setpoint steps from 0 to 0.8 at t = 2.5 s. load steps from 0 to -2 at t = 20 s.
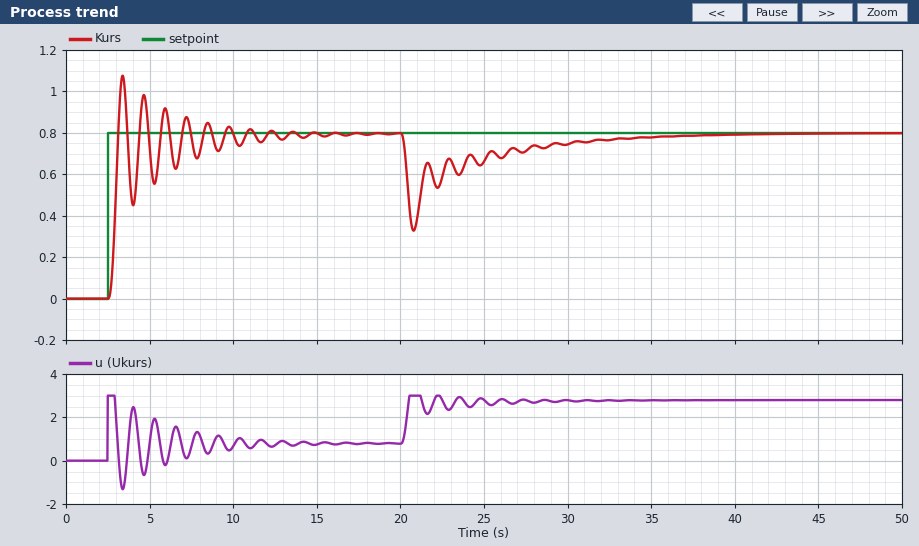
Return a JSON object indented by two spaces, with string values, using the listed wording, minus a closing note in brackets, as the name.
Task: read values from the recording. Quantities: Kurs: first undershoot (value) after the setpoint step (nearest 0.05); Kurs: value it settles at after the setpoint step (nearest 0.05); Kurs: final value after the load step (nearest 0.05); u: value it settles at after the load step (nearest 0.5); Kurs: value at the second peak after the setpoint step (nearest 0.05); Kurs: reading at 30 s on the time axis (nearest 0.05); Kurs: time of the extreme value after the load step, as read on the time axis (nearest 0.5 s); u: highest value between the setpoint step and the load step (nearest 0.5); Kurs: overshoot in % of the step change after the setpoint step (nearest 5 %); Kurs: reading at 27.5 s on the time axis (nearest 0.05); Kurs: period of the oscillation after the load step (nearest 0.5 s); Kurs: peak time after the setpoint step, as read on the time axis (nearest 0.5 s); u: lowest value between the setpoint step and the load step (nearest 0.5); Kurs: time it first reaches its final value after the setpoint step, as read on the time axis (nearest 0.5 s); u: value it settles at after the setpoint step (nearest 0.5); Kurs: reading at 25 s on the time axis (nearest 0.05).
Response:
{
  "Kurs: first undershoot (value) after the setpoint step": "0.45",
  "Kurs: value it settles at after the setpoint step": "0.80",
  "Kurs: final value after the load step": "0.80",
  "u: value it settles at after the load step": "3.0",
  "Kurs: value at the second peak after the setpoint step": "1.00",
  "Kurs: reading at 30 s on the time axis": "0.75",
  "Kurs: time of the extreme value after the load step, as read on the time axis": "21.0 s",
  "u: highest value between the setpoint step and the load step": "3.0",
  "Kurs: overshoot in % of the step change after the setpoint step": "35 %",
  "Kurs: reading at 27.5 s on the time axis": "0.70",
  "Kurs: period of the oscillation after the load step": "1.5 s",
  "Kurs: peak time after the setpoint step, as read on the time axis": "3.5 s",
  "u: lowest value between the setpoint step and the load step": "-1.5",
  "Kurs: time it first reaches its final value after the setpoint step, as read on the time axis": "3.0 s",
  "u: value it settles at after the setpoint step": "1.0",
  "Kurs: reading at 25 s on the time axis": "0.65"
}
